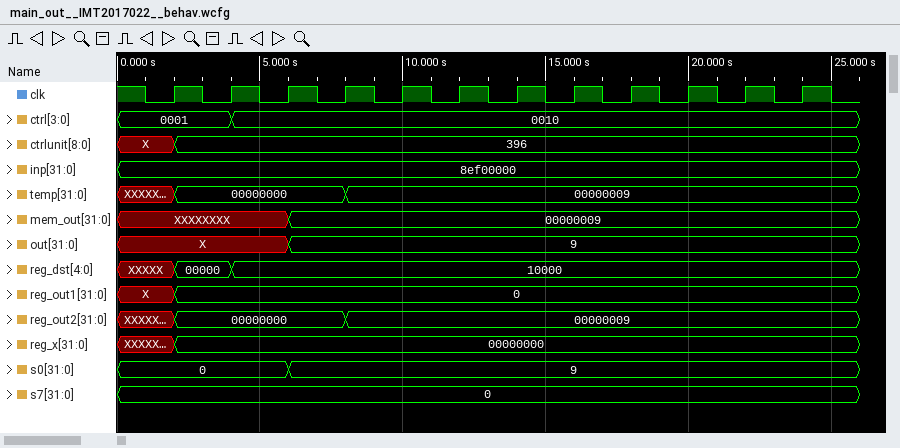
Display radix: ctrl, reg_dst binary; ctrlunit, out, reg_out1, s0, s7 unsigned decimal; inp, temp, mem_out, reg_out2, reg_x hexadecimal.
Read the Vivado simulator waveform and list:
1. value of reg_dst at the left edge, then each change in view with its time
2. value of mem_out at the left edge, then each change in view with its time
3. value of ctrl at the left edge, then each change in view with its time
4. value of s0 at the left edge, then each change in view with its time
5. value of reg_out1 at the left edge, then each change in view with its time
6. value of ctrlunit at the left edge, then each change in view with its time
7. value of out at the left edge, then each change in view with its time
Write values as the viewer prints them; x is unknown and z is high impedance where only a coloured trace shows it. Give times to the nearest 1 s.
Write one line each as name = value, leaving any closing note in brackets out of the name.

value of reg_dst at the left edge, then each change in view with its time = XXXXX, 00000 at 2 s, 10000 at 4 s
value of mem_out at the left edge, then each change in view with its time = XXXXXXXX, 00000009 at 6 s
value of ctrl at the left edge, then each change in view with its time = 0001, 0010 at 4 s
value of s0 at the left edge, then each change in view with its time = 0, 9 at 6 s
value of reg_out1 at the left edge, then each change in view with its time = X, 0 at 2 s
value of ctrlunit at the left edge, then each change in view with its time = X, 396 at 2 s
value of out at the left edge, then each change in view with its time = X, 9 at 6 s
